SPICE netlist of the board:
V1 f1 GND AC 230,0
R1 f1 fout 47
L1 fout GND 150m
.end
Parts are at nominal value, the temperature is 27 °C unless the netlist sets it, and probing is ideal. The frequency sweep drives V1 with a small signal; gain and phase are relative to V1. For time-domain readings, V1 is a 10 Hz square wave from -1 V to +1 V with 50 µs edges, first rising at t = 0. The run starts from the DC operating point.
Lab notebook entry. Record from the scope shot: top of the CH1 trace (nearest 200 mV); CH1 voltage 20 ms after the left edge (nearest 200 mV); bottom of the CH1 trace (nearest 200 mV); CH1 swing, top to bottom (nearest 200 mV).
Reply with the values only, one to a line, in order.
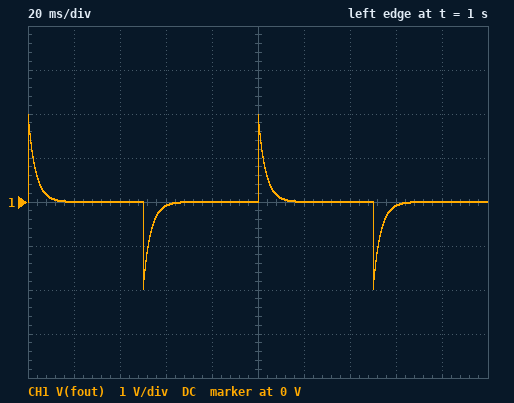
2.0 V
0 V
-2.0 V
4.0 V
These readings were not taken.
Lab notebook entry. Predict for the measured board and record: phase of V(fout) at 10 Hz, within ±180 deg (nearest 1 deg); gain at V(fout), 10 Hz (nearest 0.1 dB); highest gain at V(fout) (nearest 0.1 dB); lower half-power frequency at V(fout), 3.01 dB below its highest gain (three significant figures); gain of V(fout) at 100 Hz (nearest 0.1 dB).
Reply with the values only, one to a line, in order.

79 deg
-14.1 dB
0 dB
49.9 Hz
-1.0 dB
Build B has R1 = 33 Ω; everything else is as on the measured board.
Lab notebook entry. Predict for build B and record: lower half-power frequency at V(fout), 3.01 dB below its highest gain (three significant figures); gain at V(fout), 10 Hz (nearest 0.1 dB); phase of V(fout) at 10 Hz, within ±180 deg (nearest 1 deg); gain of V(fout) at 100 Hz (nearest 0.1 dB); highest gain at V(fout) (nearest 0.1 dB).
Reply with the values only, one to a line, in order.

35.0 Hz
-11.2 dB
74 deg
-0.5 dB
0 dB
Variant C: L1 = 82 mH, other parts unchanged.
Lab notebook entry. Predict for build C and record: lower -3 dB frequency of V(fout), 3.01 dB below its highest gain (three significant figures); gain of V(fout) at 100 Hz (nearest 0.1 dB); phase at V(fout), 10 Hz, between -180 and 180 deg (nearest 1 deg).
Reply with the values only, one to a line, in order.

91.2 Hz
-2.6 dB
84 deg
